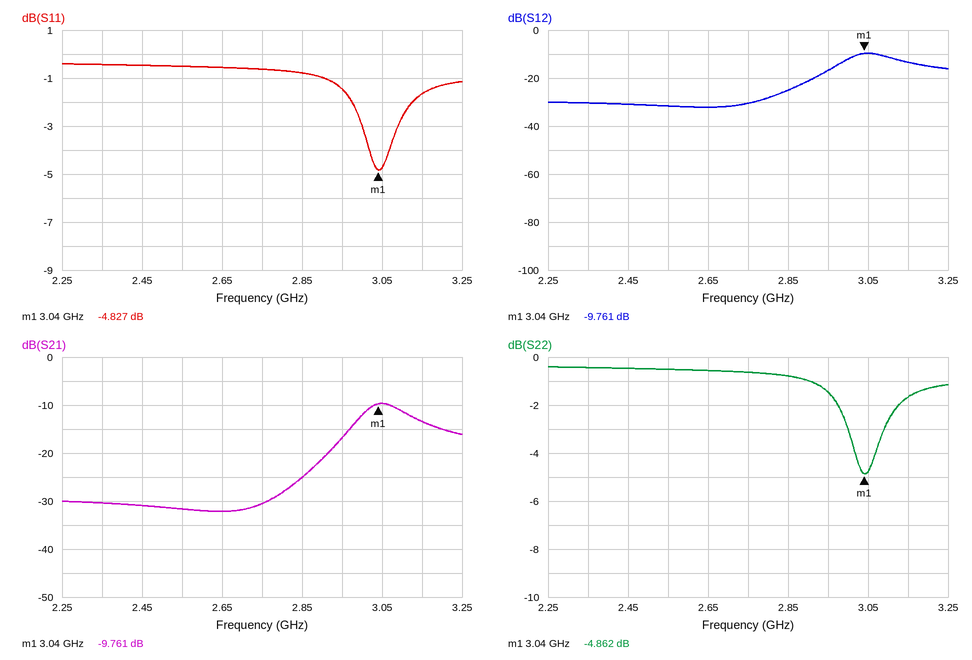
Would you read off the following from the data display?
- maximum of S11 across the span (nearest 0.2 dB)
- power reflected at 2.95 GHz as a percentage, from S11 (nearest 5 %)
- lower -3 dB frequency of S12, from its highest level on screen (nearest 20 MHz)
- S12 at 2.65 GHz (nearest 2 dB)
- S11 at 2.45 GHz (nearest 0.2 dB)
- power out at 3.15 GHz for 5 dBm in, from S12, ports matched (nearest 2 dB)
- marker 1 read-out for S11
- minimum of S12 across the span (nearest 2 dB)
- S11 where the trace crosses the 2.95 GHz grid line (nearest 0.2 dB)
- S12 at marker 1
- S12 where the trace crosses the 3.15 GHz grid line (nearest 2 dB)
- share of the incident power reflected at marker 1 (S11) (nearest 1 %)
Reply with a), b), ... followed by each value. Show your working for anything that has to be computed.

a) -0.4 dB
b) 10^(-1.4/10) ≈ 72.4 %, so 70 % to the nearest 5 %
c) 3.00 GHz
d) -32 dB
e) -0.4 dB
f) 5 dBm + (-14 dB) = -8 dBm
g) -4.827 dB
h) -32 dB
i) -1.4 dB
j) -9.761 dB
k) -14 dB
l) 10^(-4.827/10) ≈ 33 %
